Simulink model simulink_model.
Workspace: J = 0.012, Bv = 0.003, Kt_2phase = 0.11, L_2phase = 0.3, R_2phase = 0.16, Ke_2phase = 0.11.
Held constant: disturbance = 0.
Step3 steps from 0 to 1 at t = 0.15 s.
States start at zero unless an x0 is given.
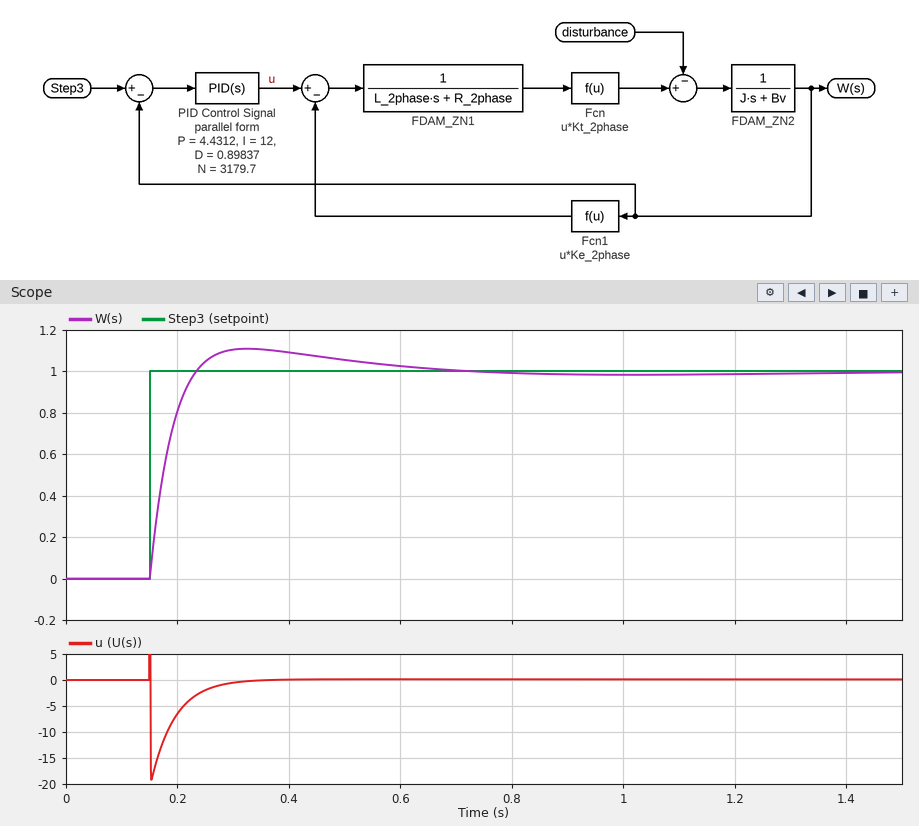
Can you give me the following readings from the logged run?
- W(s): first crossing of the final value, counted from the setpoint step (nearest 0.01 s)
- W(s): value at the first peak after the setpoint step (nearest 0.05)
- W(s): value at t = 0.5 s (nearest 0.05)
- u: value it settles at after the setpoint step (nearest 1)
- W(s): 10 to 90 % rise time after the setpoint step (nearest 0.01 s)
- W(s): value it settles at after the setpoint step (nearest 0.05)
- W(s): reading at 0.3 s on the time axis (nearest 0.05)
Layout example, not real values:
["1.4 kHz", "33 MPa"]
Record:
["0.08 s", "1.10", "1.05", "0", "0.06 s", "1.00", "1.10"]
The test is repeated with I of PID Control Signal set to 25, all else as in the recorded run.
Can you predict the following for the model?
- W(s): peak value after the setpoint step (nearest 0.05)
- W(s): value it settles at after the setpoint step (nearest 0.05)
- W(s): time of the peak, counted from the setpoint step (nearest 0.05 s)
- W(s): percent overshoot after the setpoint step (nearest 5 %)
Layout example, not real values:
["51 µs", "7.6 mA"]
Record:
["1.15", "1.00", "0.20 s", "15 %"]
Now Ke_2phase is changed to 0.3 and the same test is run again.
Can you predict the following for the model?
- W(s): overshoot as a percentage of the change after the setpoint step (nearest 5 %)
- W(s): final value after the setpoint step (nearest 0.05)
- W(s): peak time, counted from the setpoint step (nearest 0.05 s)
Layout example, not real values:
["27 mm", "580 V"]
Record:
["10 %", "1.00", "0.15 s"]
